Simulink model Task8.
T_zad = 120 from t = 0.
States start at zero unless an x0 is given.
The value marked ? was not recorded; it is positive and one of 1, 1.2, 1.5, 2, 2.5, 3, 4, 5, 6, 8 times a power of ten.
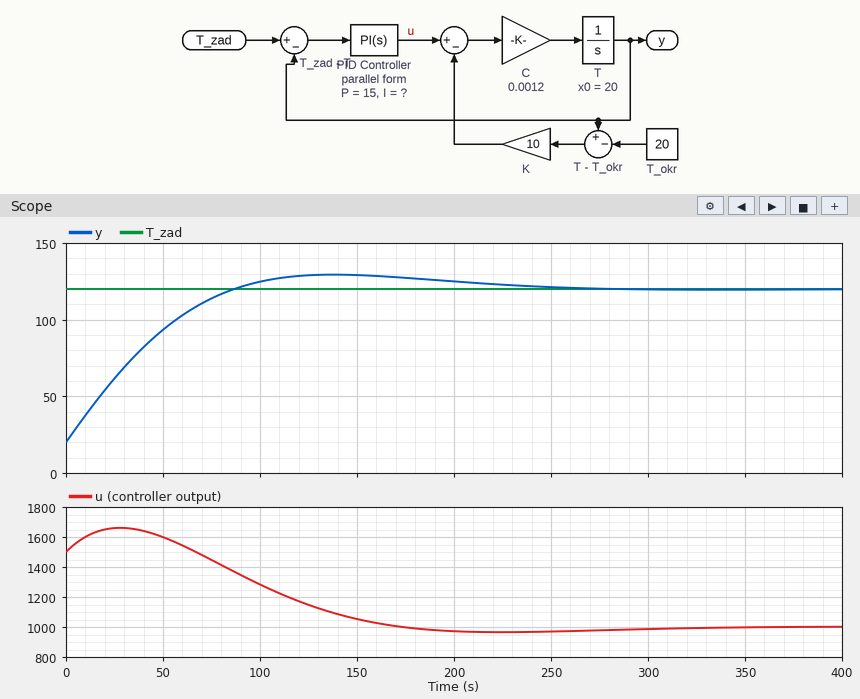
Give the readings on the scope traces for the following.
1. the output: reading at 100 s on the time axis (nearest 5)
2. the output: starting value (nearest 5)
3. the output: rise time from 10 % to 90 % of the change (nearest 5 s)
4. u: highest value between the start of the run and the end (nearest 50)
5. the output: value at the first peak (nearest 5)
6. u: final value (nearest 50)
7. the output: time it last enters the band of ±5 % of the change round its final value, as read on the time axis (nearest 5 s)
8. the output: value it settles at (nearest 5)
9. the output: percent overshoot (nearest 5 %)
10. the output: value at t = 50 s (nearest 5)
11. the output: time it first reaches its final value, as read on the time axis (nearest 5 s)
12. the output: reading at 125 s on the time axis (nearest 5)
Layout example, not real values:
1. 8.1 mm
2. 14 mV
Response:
1. 125
2. 20
3. 65 s
4. 1650
5. 130
6. 1000
7. 200 s
8. 120
9. 10 %
10. 95
11. 85 s
12. 130
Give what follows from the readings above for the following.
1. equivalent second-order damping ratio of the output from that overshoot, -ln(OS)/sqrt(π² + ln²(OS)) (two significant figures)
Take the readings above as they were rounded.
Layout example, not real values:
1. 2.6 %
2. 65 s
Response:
1. 0.59
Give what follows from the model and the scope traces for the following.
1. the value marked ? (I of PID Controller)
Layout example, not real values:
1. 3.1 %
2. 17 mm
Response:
1. 0.4
